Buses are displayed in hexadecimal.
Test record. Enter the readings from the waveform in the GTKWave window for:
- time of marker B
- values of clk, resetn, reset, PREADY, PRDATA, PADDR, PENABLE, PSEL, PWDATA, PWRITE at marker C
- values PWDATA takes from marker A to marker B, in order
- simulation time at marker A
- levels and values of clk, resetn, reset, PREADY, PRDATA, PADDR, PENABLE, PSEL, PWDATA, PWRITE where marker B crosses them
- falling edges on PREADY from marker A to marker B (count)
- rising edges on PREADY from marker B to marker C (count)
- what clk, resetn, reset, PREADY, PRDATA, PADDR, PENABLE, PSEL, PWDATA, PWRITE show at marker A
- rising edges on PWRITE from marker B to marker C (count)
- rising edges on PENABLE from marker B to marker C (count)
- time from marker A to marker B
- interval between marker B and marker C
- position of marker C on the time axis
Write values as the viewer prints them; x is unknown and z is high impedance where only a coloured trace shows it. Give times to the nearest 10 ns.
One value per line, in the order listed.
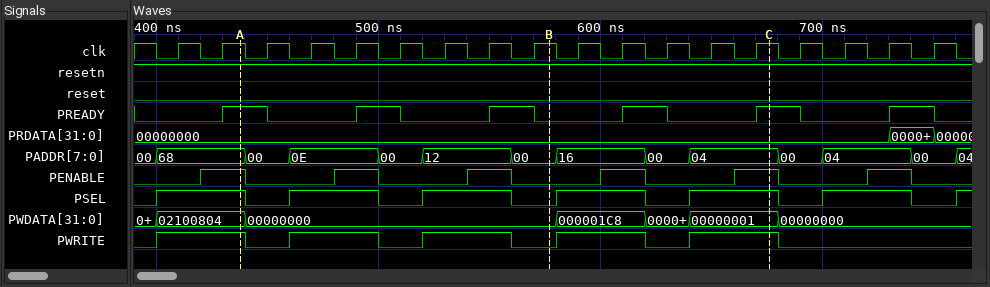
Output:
580 ns
clk=1, resetn=1, reset=0, PREADY=1, PRDATA=00000000, PADDR=04, PENABLE=1, PSEL=1, PWDATA=00000001, PWRITE=1
02100804, 00000000
440 ns
clk=1, resetn=1, reset=0, PREADY=0, PRDATA=00000000, PADDR=00, PENABLE=0, PSEL=0, PWDATA=00000000, PWRITE=0
3
2
clk=1, resetn=1, reset=0, PREADY=1, PRDATA=00000000, PADDR=68, PENABLE=1, PSEL=1, PWDATA=02100804, PWRITE=1
2
2
140 ns
100 ns
680 ns
